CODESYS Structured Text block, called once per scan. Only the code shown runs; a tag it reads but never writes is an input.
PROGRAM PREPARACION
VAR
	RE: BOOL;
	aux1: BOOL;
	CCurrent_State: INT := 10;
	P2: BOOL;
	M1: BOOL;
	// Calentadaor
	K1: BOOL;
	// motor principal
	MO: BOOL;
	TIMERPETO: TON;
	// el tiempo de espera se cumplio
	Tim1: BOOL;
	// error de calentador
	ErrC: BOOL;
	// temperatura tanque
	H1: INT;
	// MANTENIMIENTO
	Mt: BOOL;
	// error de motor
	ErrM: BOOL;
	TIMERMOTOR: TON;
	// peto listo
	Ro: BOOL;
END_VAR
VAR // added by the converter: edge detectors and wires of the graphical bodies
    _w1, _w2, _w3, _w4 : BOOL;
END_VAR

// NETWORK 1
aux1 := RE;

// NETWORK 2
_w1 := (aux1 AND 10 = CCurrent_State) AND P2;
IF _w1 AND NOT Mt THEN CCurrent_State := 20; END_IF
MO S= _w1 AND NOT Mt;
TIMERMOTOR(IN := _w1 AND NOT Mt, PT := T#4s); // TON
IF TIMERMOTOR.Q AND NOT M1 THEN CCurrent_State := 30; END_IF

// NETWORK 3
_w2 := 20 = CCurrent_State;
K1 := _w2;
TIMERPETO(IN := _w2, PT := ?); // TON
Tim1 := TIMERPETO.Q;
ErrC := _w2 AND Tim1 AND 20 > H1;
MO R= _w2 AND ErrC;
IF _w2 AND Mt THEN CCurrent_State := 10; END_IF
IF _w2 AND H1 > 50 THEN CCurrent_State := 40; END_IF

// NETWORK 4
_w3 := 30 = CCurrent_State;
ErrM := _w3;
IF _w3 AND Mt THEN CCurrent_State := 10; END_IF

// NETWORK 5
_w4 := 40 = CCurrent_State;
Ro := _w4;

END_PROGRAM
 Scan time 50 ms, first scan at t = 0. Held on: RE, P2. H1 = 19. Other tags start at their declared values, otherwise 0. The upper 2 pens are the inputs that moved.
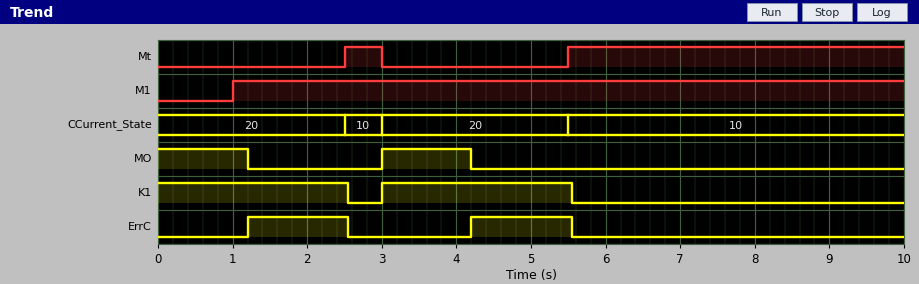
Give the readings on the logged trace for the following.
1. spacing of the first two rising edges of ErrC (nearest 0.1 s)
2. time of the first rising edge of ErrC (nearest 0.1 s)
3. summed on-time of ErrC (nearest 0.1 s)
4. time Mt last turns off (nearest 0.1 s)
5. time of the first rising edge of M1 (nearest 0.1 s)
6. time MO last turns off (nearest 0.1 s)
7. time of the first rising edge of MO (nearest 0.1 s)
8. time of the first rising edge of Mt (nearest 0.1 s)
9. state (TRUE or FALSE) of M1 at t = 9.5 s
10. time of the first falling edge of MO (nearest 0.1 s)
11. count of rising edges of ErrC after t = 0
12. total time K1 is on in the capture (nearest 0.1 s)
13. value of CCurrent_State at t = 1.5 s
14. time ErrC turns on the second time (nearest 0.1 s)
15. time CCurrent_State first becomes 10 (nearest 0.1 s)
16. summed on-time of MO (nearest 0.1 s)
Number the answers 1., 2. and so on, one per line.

1. 3.0 s
2. 1.2 s
3. 2.7 s
4. 3.0 s
5. 1.0 s
6. 4.2 s
7. 3.0 s
8. 2.5 s
9. TRUE
10. 1.2 s
11. 2
12. 5.1 s
13. 20
14. 4.2 s
15. 2.5 s
16. 2.4 s
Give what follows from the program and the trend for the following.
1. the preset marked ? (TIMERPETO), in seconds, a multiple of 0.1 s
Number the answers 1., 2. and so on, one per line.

1. 1.2 s
